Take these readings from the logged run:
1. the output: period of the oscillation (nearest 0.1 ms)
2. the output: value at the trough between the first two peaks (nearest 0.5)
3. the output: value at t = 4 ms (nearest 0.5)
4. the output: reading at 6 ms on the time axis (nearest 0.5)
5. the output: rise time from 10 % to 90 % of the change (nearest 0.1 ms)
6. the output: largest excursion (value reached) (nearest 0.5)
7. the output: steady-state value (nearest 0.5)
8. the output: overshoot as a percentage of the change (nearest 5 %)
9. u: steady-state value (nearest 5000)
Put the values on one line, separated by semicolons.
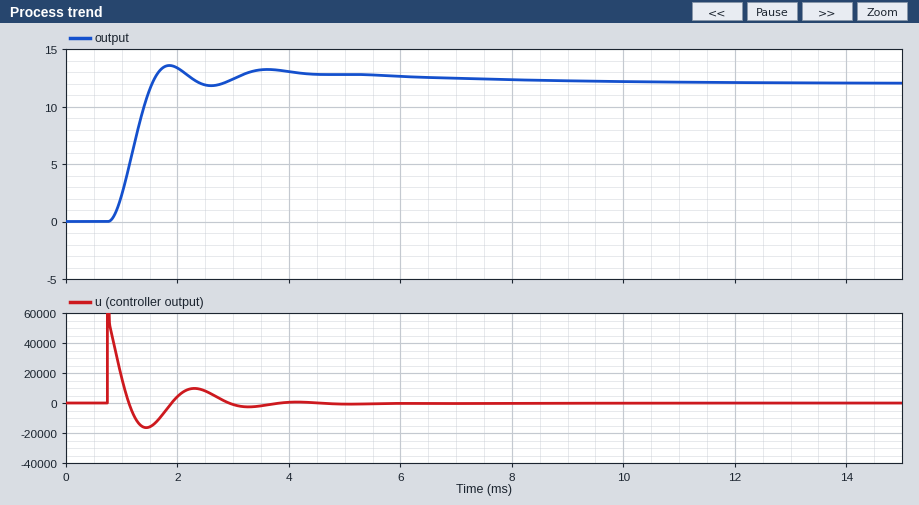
1.8 ms; 12.0; 13.0; 12.5; 0.5 ms; 13.5; 12.0; 15 %; 0
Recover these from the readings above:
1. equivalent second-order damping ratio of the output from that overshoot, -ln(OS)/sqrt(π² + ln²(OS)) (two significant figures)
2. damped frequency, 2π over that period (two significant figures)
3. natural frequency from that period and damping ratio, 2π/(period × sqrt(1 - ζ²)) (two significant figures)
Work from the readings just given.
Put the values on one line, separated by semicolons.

0.52; 3.5 rad/ms; 4.1 rad/ms
